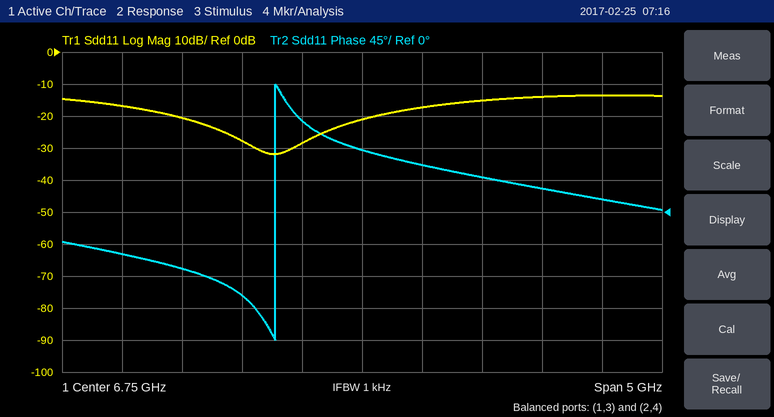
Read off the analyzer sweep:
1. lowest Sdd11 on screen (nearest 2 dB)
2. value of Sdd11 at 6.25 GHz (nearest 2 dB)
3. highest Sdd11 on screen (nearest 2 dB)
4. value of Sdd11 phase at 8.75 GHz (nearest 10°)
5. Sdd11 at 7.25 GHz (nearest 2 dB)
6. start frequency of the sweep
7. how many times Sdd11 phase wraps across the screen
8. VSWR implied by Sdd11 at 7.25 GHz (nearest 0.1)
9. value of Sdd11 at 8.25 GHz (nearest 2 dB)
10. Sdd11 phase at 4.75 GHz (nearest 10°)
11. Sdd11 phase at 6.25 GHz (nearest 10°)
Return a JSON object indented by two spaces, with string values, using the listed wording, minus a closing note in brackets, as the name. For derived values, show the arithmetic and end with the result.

{
  "lowest Sdd11 on screen": "-32 dB",
  "value of Sdd11 at 6.25 GHz": "-28 dB",
  "highest Sdd11 on screen": "-14 dB",
  "value of Sdd11 phase at 8.75 GHz": "20°",
  "Sdd11 at 7.25 GHz": "-18 dB",
  "start frequency of the sweep": "4.25 GHz",
  "how many times Sdd11 phase wraps across the screen": "1",
  "VSWR implied by Sdd11 at 7.25 GHz": "|Γ| = 10^(-18/20) = 0.1259; VSWR = (1 + 0.1259)/(1 − 0.1259) ≈ 1.3",
  "value of Sdd11 at 8.25 GHz": "-14 dB",
  "Sdd11 phase at 4.75 GHz": "-60°",
  "Sdd11 phase at 6.25 GHz": "130°"
}
